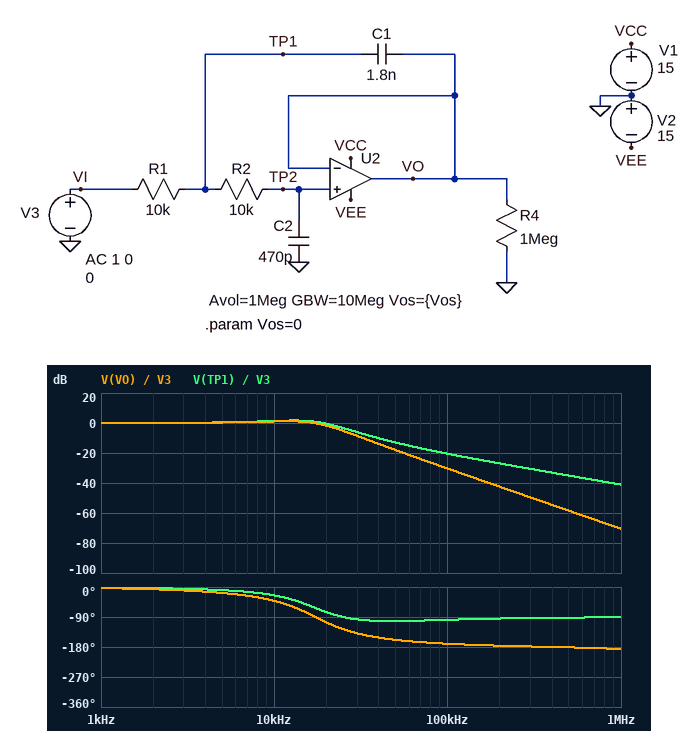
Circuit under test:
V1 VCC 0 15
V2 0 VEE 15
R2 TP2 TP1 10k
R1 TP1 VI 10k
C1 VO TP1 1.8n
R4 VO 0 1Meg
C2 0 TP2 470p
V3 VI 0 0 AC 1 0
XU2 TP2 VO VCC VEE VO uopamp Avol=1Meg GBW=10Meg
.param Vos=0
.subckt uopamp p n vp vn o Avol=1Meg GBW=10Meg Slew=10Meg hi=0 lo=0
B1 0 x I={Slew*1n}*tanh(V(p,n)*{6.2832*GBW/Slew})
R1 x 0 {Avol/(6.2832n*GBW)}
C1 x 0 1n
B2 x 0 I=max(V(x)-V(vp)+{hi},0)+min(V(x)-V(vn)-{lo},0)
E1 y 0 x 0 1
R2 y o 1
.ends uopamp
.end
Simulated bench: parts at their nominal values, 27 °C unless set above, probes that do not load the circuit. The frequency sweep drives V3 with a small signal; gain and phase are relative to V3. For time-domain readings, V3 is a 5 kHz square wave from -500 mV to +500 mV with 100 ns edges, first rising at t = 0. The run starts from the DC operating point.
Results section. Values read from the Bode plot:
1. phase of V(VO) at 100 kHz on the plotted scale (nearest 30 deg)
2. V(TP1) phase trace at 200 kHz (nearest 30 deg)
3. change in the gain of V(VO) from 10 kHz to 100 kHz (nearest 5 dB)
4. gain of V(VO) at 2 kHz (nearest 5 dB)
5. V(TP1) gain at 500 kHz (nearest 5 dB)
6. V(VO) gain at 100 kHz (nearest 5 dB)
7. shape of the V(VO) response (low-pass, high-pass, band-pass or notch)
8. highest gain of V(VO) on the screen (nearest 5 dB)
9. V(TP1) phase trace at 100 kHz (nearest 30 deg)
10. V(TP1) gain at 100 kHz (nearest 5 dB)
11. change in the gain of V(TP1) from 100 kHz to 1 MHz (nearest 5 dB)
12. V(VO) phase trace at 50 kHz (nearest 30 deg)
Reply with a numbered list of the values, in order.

1. -180 deg
2. -90 deg
3. -30 dB
4. 0 dB
5. -35 dB
6. -30 dB
7. low-pass
8. 0 dB
9. -90 deg
10. -20 dB
11. -20 dB
12. -150 deg
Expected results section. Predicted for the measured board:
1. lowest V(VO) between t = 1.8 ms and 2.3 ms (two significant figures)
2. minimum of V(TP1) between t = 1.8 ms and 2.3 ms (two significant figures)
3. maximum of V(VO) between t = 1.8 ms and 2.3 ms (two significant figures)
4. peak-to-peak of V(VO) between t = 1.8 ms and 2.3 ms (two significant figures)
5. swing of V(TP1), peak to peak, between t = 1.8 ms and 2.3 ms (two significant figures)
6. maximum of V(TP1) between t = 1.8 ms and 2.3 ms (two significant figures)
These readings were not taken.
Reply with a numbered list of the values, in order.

1. -660 mV
2. -680 mV
3. 660 mV
4. 1.3 V
5. 1.4 V
6. 680 mV
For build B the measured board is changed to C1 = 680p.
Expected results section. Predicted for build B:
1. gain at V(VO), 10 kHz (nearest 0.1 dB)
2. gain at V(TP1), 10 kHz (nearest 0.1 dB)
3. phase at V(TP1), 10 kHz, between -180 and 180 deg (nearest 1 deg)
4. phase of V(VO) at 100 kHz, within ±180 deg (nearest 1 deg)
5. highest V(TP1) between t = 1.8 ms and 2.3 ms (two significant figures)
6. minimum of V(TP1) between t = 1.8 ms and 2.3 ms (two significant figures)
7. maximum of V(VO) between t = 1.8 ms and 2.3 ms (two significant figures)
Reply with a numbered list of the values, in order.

1. -0.5 dB
2. -0.1 dB
3. -18 deg
4. -154 deg
5. 520 mV
6. -520 mV
7. 510 mV
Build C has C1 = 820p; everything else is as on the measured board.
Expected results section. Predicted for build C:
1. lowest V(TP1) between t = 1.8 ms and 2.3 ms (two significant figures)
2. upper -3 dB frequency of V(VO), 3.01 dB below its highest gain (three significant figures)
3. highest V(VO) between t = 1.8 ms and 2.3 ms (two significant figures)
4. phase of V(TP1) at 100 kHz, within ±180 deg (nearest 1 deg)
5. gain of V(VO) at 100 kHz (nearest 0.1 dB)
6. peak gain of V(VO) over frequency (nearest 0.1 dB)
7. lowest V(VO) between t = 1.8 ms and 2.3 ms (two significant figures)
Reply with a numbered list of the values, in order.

1. -550 mV
2. 23.8 kHz
3. 530 mV
4. -86 deg
5. -23.8 dB
6. 0 dB
7. -530 mV
